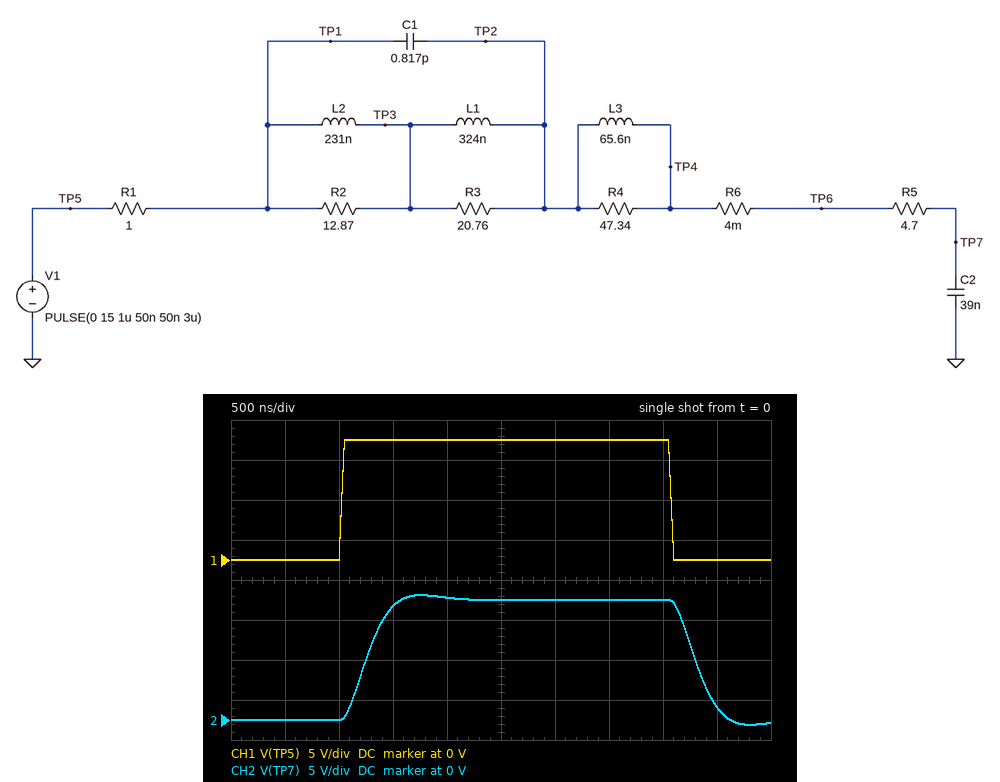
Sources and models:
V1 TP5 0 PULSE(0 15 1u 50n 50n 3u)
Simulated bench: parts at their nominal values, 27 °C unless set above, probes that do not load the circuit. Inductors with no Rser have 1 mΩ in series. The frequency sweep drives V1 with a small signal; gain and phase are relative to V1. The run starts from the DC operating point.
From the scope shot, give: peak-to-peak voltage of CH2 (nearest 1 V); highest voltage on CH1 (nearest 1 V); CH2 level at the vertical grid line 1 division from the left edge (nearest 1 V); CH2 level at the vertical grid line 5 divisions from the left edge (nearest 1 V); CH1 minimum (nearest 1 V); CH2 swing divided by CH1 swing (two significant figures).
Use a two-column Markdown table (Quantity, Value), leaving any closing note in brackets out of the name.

| Quantity | Value |
|---|---|
| peak-to-peak voltage of CH2 | 16 V |
| highest voltage on CH1 | 15 V |
| CH2 level at the vertical grid line 1 division from the left edge | 0 V |
| CH2 level at the vertical grid line 5 divisions from the left edge | 15 V |
| CH1 minimum | 0 V |
| CH2 swing divided by CH1 swing | 1.1 |
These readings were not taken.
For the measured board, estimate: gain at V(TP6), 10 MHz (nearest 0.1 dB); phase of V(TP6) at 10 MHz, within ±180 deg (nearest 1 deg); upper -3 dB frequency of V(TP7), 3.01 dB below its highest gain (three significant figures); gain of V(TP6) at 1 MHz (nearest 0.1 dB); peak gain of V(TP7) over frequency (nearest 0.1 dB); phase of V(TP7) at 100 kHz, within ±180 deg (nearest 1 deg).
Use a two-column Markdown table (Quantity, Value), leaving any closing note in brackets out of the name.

| Quantity | Value |
|---|---|
| gain at V(TP6), 10 MHz | -16.4 dB |
| phase of V(TP6) at 10 MHz, within ±180 deg | -46 deg |
| upper -3 dB frequency of V(TP7), 3.01 dB below its highest gain | 951 kHz |
| gain of V(TP6) at 1 MHz | 0.2 dB |
| peak gain of V(TP7) over frequency | 0 dB |
| phase of V(TP7) at 100 kHz, within ±180 deg | -8 deg |
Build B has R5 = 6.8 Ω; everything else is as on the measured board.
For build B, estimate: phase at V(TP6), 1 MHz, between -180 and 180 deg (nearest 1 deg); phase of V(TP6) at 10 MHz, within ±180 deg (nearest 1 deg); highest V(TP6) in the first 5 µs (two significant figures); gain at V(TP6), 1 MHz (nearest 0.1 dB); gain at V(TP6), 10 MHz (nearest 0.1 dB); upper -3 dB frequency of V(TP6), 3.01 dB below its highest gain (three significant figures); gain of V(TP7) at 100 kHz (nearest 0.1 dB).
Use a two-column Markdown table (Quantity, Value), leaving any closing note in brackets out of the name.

| Quantity | Value |
|---|---|
| phase at V(TP6), 1 MHz, between -180 and 180 deg | -29 deg |
| phase of V(TP6) at 10 MHz, within ±180 deg | -42 deg |
| highest V(TP6) in the first 5 µs | 16 V |
| gain at V(TP6), 1 MHz | -0.3 dB |
| gain at V(TP6), 10 MHz | -13.6 dB |
| upper -3 dB frequency of V(TP6), 3.01 dB below its highest gain | 1.68 MHz |
| gain of V(TP7) at 100 kHz | -0.1 dB |
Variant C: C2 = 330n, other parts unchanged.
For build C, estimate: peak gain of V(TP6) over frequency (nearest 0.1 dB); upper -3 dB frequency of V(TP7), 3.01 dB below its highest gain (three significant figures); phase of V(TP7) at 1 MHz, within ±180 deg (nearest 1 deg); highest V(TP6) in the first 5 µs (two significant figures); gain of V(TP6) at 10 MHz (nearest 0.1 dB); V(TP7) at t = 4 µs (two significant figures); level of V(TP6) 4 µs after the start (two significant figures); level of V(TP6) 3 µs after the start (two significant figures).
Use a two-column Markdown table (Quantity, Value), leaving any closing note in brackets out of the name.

| Quantity | Value |
|---|---|
| peak gain of V(TP6) over frequency | 0 dB |
| upper -3 dB frequency of V(TP7), 3.01 dB below its highest gain | 89.6 kHz |
| phase of V(TP7) at 1 MHz, within ±180 deg | -119 deg |
| highest V(TP6) in the first 5 µs | 15 V |
| gain of V(TP6) at 10 MHz | -16.5 dB |
| V(TP7) at t = 4 µs | 12 V |
| level of V(TP6) 4 µs after the start | 15 V |
| level of V(TP6) 3 µs after the start | 14 V |
